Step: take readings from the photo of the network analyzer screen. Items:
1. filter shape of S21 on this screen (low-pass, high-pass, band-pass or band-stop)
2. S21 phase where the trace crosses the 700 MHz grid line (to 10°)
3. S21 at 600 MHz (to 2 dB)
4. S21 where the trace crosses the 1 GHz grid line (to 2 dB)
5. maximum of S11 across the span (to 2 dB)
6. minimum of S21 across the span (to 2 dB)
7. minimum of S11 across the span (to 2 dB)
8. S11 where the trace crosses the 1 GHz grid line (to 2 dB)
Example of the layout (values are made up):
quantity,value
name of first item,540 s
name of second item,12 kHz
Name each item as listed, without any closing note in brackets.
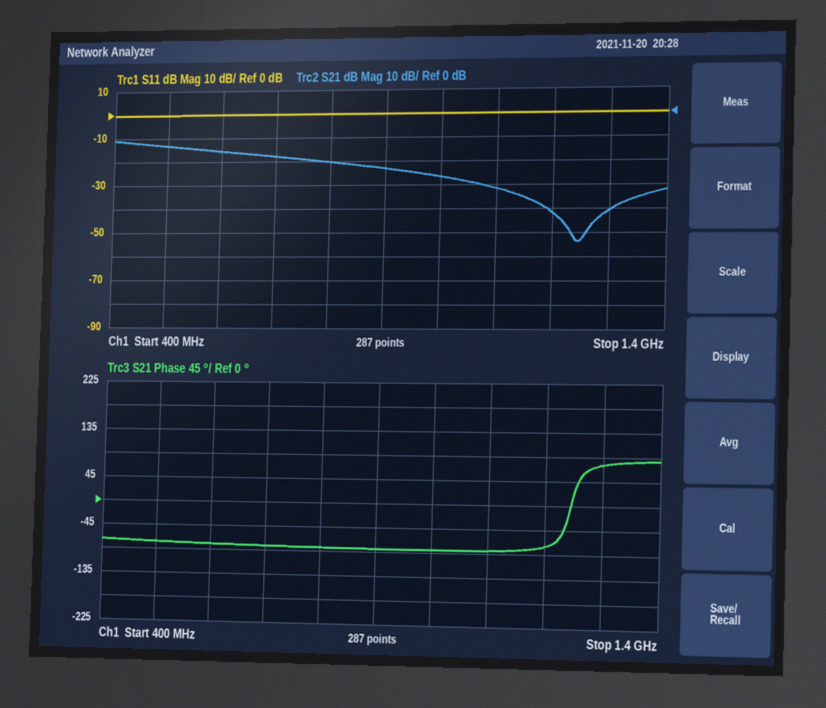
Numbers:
quantity,value
filter shape of S21 on this screen,low-pass
S21 phase where the trace crosses the 700 MHz grid line,-80°
S21 at 600 MHz,-16 dB
S21 where the trace crosses the 1 GHz grid line,-26 dB
maximum of S11 across the span,0 dB
minimum of S21 across the span,-54 dB
minimum of S11 across the span,0 dB
S11 where the trace crosses the 1 GHz grid line,0 dB
